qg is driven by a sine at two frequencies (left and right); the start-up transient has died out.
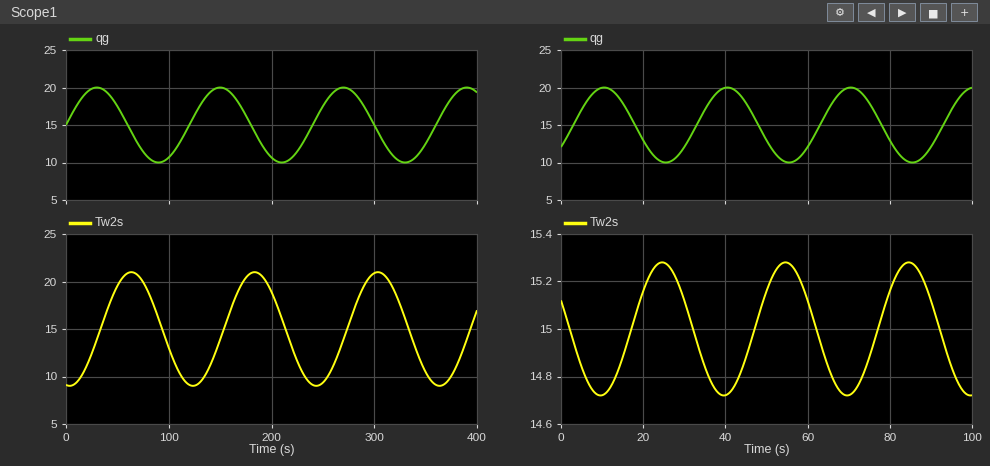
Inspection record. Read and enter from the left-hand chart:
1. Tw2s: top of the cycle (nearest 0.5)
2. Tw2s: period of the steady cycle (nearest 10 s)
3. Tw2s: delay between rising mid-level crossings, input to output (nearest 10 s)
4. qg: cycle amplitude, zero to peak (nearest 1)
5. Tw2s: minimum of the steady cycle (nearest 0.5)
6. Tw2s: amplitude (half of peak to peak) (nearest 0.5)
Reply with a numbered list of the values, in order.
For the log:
1. 21.0
2. 120 s
3. 30 s
4. 5
5. 9.0
6. 6.0
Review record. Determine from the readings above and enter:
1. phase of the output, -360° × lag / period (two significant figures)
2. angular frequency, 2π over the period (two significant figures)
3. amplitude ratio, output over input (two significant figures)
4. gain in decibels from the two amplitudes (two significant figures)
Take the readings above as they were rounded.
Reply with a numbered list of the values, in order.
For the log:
1. -90°
2. 0.052 rad/s
3. 1.2
4. 1.6 dB
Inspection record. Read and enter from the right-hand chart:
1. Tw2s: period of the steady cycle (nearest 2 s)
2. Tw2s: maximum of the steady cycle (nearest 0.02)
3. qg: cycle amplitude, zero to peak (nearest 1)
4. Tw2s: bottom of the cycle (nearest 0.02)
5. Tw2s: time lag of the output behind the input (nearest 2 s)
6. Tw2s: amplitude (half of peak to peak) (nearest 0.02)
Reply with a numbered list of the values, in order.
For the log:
1. 30 s
2. 15.28
3. 5
4. 14.72
5. 14 s
6. 0.28
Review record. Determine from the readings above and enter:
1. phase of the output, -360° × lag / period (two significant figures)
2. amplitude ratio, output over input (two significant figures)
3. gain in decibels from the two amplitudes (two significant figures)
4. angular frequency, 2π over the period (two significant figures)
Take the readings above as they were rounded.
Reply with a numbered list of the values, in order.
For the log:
1. -170°
2. 0.056
3. -25 dB
4. 0.21 rad/s
